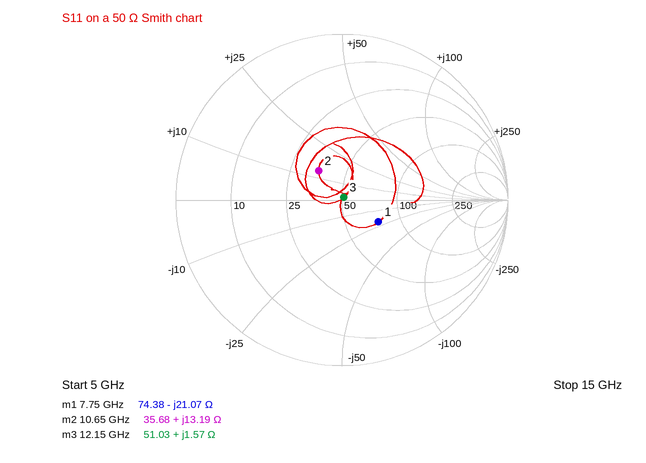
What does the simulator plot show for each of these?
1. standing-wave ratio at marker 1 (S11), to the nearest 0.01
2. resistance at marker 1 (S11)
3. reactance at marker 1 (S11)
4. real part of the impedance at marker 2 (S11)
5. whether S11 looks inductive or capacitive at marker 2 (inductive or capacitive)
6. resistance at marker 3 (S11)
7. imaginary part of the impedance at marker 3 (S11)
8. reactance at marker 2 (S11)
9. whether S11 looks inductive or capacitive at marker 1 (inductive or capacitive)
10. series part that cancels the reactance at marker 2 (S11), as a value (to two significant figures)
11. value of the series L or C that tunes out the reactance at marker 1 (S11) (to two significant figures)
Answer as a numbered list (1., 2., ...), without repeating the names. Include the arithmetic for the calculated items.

1. 1.69
2. 74.38 Ω
3. -21.07 Ω
4. 35.68 Ω
5. inductive
6. 51.03 Ω
7. +1.57 Ω
8. +13.19 Ω
9. capacitive
10. C = 1/(2π × 10.65 GHz × 13.19 Ω) ≈ 1.1 pF
11. L = 21.07 Ω/(2π × 7.75 GHz) ≈ 433 pH, so 430 pH to two significant figures
